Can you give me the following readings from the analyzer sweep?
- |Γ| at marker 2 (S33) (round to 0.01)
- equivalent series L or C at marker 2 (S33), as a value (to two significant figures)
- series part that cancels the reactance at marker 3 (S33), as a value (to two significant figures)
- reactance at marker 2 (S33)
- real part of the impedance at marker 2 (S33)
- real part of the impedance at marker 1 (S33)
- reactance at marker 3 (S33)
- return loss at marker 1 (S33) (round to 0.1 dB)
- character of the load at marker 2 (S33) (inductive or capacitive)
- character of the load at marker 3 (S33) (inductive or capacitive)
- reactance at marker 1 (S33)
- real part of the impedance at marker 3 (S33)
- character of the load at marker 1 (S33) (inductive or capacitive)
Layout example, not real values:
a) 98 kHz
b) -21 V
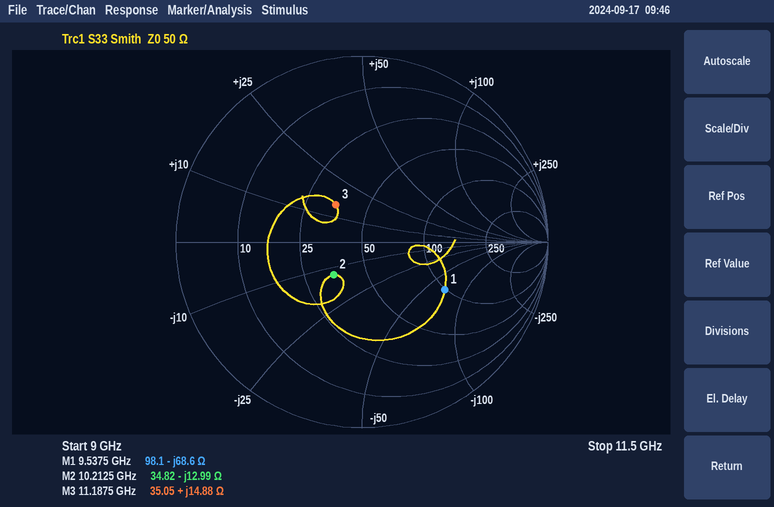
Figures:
a) 0.23
b) 1.2 pF
c) 960 fF
d) -12.99 Ω
e) 34.82 Ω
f) 98.1 Ω
g) +14.88 Ω
h) 5.8 dB
i) capacitive
j) inductive
k) -68.6 Ω
l) 35.05 Ω
m) capacitive
